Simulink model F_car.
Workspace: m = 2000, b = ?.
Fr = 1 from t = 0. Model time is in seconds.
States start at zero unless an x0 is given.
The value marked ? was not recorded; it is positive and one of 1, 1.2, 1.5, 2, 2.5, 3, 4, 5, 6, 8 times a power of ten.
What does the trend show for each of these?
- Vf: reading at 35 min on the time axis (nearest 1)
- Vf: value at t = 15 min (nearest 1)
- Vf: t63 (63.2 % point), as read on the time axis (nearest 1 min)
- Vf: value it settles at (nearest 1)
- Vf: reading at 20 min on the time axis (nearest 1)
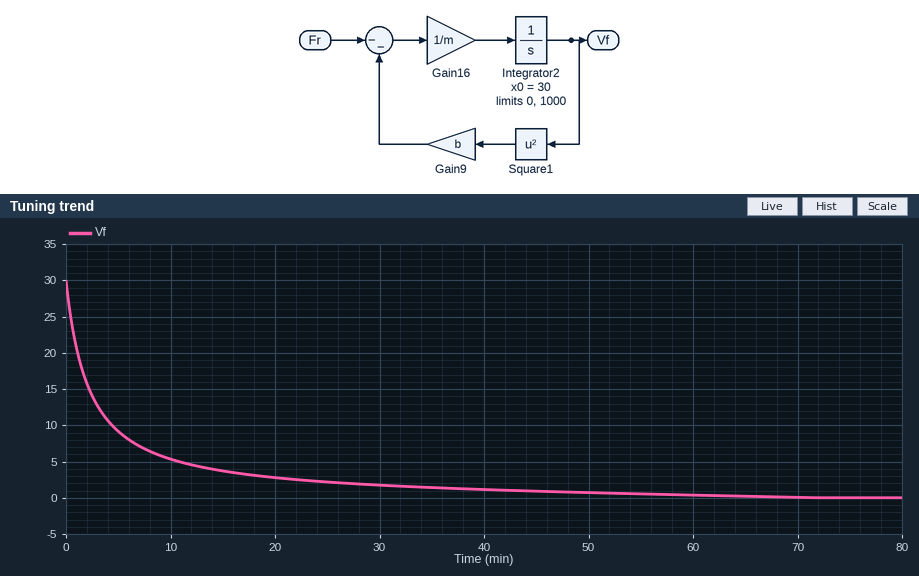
1
4
4 min
0
3
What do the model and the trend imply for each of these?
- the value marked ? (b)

0.5
